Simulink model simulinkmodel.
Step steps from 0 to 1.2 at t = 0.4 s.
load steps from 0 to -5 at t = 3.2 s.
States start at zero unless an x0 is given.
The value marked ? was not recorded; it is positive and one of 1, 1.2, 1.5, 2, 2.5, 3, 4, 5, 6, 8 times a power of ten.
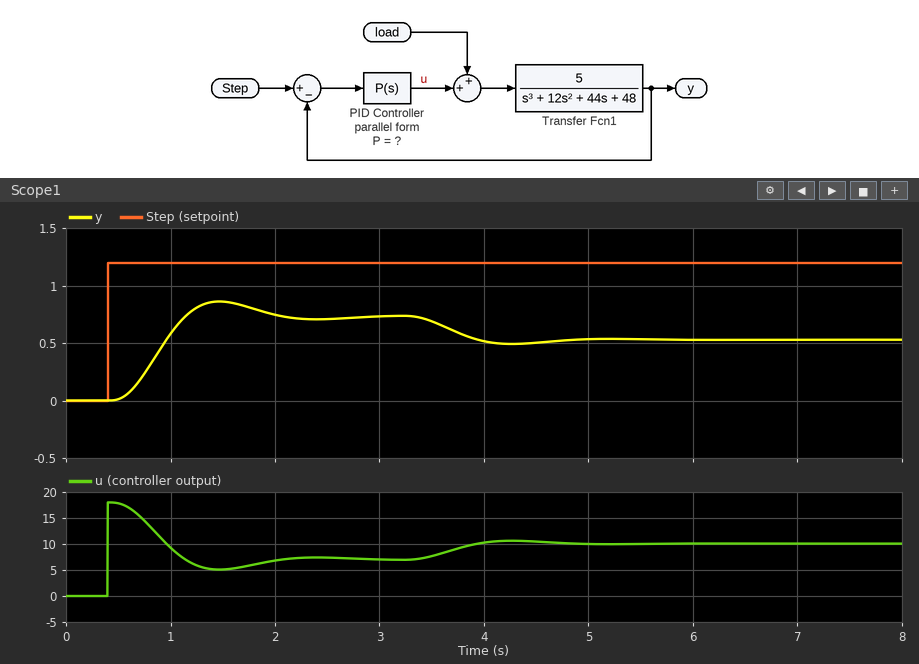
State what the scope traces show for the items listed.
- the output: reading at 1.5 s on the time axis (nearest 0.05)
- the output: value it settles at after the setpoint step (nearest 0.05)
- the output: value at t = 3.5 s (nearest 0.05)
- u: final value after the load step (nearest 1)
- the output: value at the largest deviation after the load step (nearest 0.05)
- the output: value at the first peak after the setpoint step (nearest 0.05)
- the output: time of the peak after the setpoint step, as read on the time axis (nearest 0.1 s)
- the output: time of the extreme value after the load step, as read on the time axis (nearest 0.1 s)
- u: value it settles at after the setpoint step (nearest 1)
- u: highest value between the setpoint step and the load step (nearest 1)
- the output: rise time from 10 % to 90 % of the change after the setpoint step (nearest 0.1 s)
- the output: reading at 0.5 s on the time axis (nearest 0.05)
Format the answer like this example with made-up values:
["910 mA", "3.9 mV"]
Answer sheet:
["0.85", "0.75", "0.70", "10", "0.50", "0.85", "1.5 s", "4.3 s", "7", "18", "0.5 s", "0.00"]
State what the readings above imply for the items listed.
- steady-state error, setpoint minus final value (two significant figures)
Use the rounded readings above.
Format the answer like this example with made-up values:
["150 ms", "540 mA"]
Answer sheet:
["0.45"]
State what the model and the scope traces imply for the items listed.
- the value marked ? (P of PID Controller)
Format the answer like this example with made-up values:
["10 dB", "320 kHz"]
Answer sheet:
["15"]
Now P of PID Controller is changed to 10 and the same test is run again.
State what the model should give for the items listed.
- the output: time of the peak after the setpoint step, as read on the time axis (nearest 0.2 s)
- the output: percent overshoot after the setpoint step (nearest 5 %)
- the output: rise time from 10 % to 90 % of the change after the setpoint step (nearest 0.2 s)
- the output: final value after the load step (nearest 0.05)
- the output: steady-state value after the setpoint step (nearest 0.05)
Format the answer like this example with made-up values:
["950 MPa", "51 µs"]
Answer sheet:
["1.6 s", "10 %", "0.6 s", "0.35", "0.60"]
